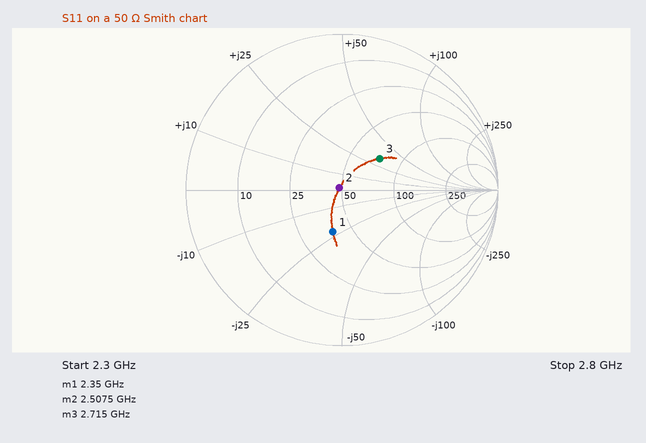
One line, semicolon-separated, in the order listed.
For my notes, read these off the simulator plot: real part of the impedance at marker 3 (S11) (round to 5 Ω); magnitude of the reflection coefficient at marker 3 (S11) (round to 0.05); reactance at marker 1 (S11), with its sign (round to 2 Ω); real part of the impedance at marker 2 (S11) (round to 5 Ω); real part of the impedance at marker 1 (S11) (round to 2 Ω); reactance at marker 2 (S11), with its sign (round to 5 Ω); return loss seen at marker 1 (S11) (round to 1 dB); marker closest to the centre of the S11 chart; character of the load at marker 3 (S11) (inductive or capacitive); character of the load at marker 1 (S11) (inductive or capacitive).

75 Ω; 0.30; -22 Ω; 50 Ω; 38 Ω; 0 Ω; 11 dB; marker 2; inductive; capacitive
